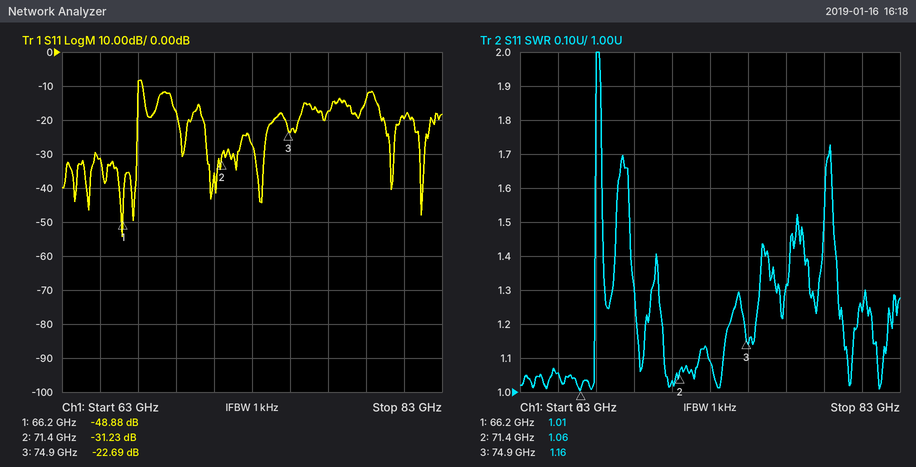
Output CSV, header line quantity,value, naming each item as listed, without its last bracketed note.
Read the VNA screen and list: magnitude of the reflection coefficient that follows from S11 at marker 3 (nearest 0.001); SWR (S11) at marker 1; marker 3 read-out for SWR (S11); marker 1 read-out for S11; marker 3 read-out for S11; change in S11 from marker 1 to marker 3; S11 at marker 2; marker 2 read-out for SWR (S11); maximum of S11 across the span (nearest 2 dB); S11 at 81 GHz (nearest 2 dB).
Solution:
quantity,value
magnitude of the reflection coefficient that follows from S11 at marker 3,0.073
SWR (S11) at marker 1,1.01
marker 3 read-out for SWR,1.16
marker 1 read-out for S11,-48.88 dB
marker 3 read-out for S11,-22.69 dB
change in S11 from marker 1 to marker 3,26.19 dB
S11 at marker 2,-31.23 dB
marker 2 read-out for SWR,1.06
maximum of S11 across the span,-8 dB
S11 at 81 GHz,-20 dB
